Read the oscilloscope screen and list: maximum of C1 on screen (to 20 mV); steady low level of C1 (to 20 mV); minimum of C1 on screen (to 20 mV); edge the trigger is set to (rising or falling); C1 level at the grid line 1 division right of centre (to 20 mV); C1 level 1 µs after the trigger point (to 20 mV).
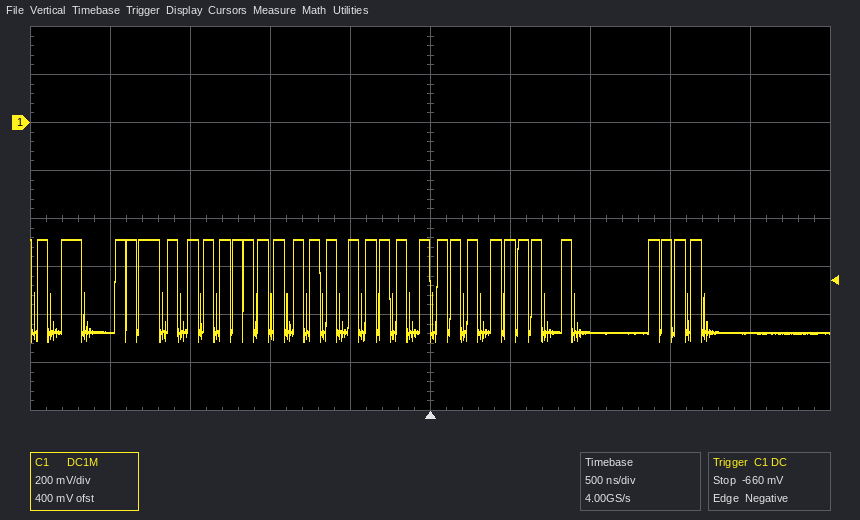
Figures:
-480 mV
-880 mV
-920 mV
falling
-480 mV
-880 mV
